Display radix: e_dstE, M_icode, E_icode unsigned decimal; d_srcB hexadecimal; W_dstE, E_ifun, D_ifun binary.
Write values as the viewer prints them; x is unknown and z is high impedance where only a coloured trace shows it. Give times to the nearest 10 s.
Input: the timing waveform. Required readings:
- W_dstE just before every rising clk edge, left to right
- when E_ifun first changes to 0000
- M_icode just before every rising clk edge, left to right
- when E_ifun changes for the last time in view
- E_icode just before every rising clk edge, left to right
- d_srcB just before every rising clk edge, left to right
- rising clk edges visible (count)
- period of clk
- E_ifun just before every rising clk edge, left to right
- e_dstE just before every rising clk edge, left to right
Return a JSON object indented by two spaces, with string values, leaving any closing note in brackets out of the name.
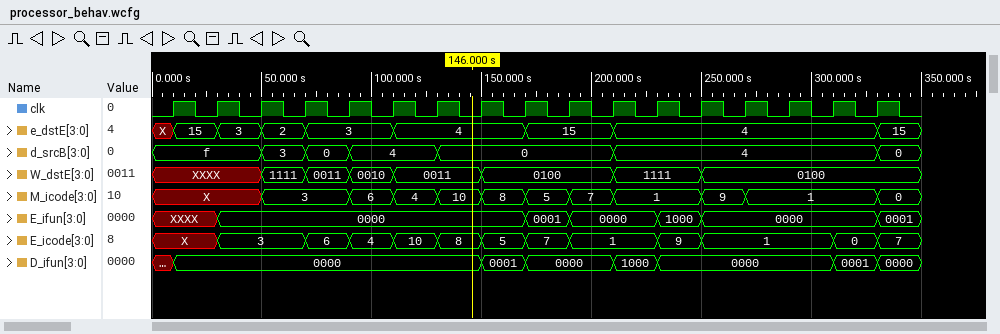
{
  "W_dstE just before every rising clk edge, left to right": "XXXX, XXXX, XXXX, 1111, 0011, 0010, 0011, 0011, 0100, 0100, 0100, 1111, 1111, 0100, 0100, 0100, 0100",
  "when E_ifun first changes to 0000": "30 s",
  "M_icode just before every rising clk edge, left to right": "X, X, X, 3, 3, 6, 4, 10, 8, 5, 7, 1, 1, 9, 1, 1, 1",
  "when E_ifun changes for the last time in view": "330 s",
  "E_icode just before every rising clk edge, left to right": "X, X, 3, 3, 6, 4, 10, 8, 5, 7, 1, 1, 9, 1, 1, 1, 0",
  "d_srcB just before every rising clk edge, left to right": "f, f, f, 3, 0, 4, 4, 0, 0, 0, 0, 4, 4, 4, 4, 4, 4",
  "rising clk edges visible": "17",
  "period of clk": "20 s",
  "E_ifun just before every rising clk edge, left to right": "XXXX, XXXX, 0000, 0000, 0000, 0000, 0000, 0000, 0000, 0001, 0000, 0000, 1000, 0000, 0000, 0000, 0000",
  "e_dstE just before every rising clk edge, left to right": "X, 15, 3, 2, 3, 3, 4, 4, 4, 15, 15, 4, 4, 4, 4, 4, 4"
}
